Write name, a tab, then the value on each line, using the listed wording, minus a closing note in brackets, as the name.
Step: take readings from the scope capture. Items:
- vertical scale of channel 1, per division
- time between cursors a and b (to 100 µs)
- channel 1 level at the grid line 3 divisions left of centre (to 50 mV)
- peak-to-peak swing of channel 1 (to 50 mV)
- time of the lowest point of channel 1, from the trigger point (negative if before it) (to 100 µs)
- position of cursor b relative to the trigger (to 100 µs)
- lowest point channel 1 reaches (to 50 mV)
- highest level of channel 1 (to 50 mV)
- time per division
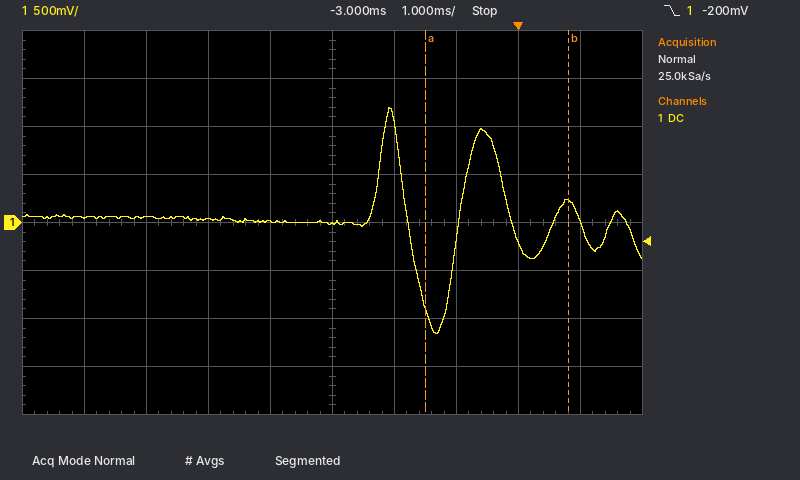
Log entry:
vertical scale of channel 1, per division	500 mV
time between cursors a and b	2.3 ms
channel 1 level at the grid line 3 divisions left of centre	50 mV
peak-to-peak swing of channel 1	2.35 V
time of the lowest point of channel 1, from the trigger point (negative if before it)	-1.3 ms
position of cursor b relative to the trigger	+800 µs
lowest point channel 1 reaches	-1.15 V
highest level of channel 1	1.20 V
time per division	1 ms
